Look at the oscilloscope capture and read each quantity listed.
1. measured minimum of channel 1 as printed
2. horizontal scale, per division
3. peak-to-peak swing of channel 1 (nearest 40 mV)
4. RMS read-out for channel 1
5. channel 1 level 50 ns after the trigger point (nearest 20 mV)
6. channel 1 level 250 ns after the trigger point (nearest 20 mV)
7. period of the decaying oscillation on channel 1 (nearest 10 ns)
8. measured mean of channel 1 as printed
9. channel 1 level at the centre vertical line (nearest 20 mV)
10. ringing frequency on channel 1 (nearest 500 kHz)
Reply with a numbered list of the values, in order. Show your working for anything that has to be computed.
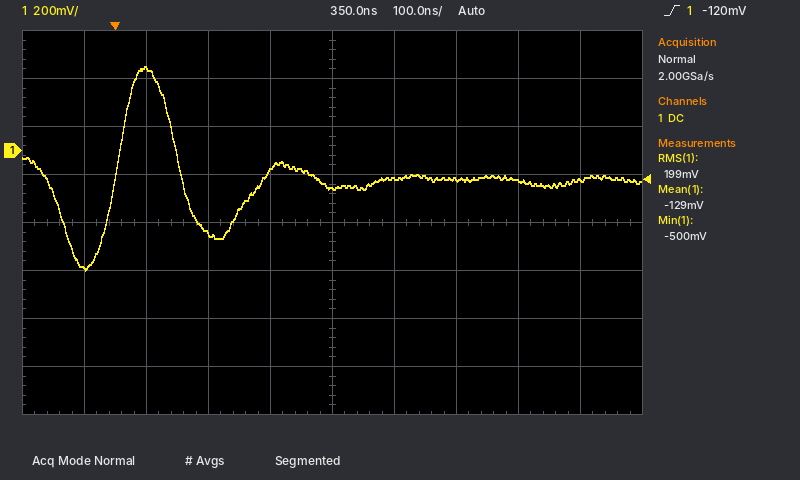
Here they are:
1. -500 mV
2. 100 ns
3. 840 mV
4. 199 mV
5. 340 mV
6. -80 mV
7. 220 ns
8. -129 mV
9. -160 mV
10. 1 / 220 ns ≈ 4.5 MHz
